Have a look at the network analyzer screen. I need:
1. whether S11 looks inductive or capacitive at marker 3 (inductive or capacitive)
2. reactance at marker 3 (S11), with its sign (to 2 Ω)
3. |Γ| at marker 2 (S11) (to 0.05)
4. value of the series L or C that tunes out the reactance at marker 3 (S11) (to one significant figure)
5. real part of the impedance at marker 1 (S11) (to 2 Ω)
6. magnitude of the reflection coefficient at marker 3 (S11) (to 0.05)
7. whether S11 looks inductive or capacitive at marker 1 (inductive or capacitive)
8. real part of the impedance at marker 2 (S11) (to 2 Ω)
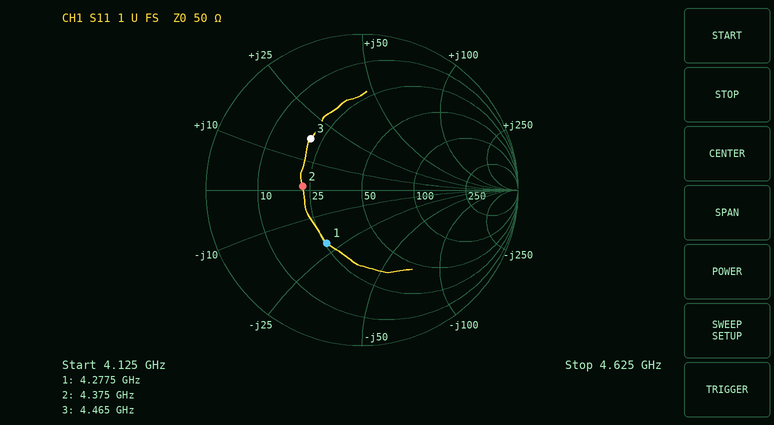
inductive
+18 Ω
0.40
2 pF
26 Ω
0.45
capacitive
22 Ω
